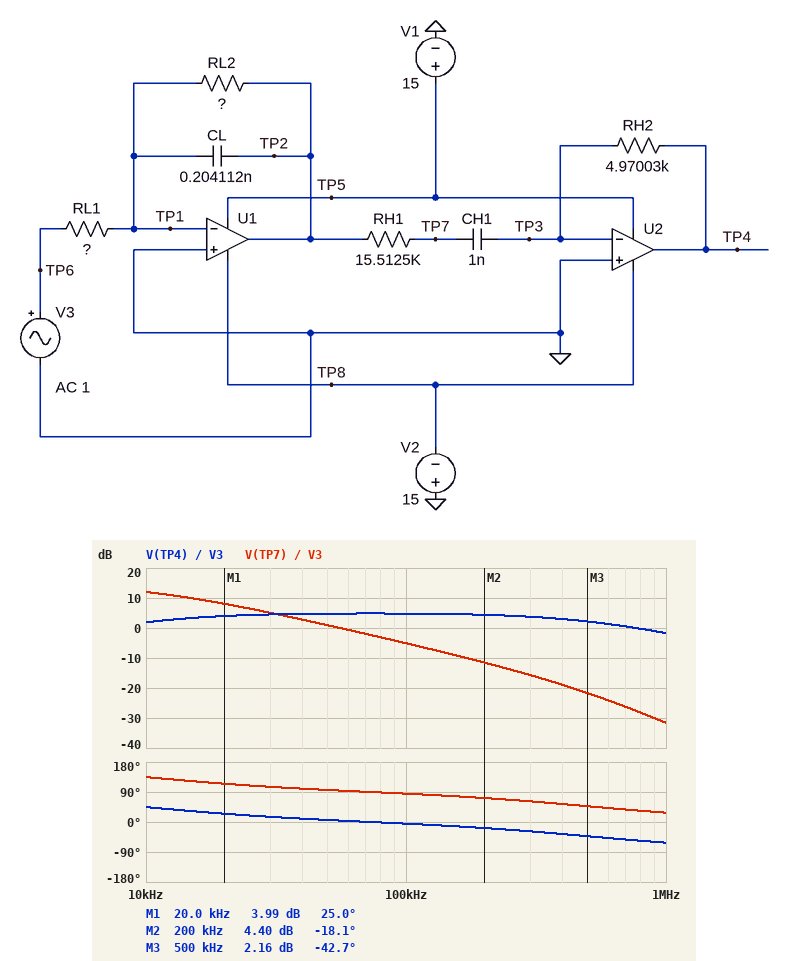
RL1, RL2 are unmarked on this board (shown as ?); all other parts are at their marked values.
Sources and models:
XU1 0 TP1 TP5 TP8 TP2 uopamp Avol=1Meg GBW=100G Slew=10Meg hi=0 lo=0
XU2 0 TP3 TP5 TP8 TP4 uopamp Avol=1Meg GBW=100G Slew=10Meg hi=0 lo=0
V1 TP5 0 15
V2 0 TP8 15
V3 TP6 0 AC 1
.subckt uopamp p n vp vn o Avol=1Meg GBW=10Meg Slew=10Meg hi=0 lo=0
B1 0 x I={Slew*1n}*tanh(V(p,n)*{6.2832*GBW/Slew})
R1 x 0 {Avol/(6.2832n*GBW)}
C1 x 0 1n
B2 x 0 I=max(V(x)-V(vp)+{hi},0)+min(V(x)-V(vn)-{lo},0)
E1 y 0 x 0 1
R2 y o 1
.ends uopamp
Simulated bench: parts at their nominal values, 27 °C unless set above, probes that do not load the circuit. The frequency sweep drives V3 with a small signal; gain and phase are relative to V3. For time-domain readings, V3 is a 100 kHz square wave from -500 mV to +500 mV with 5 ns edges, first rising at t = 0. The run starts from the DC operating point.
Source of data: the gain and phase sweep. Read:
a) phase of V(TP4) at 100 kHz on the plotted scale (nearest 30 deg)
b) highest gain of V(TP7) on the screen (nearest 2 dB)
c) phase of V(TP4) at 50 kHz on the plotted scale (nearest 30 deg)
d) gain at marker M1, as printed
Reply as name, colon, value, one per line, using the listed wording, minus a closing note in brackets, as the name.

phase of V(TP4) at 100 kHz on the plotted scale: 0 deg
highest gain of V(TP7) on the screen: 12 dB
phase of V(TP4) at 50 kHz on the plotted scale: 0 deg
gain at marker M1, as printed: 3.99 dB
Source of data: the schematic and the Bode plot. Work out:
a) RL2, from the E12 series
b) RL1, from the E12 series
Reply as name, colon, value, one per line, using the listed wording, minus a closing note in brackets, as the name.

RL2, from the E12 series: 1.5 kΩ
RL1, from the E12 series: 270 Ω
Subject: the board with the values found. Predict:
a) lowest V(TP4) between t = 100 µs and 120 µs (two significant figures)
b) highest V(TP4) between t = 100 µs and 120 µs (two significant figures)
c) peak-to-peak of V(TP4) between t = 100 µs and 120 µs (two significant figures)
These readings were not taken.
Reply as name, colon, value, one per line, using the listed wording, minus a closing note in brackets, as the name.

lowest V(TP4) between t = 100 µs and 120 µs: -940 mV
highest V(TP4) between t = 100 µs and 120 µs: 940 mV
peak-to-peak of V(TP4) between t = 100 µs and 120 µs: 1.9 V
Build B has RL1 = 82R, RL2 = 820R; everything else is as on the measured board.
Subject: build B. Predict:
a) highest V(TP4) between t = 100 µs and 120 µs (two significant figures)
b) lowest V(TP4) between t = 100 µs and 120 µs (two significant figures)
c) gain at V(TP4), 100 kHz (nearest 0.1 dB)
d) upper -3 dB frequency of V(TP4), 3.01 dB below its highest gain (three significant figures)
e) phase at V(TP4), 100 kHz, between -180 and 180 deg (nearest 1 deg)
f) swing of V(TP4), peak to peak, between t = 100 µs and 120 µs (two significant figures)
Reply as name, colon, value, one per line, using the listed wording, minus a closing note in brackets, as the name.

highest V(TP4) between t = 100 µs and 120 µs: 1.7 V
lowest V(TP4) between t = 100 µs and 120 µs: -1.7 V
gain at V(TP4), 100 kHz: 10.0 dB
upper -3 dB frequency of V(TP4), 3.01 dB below its highest gain: 971 kHz
phase at V(TP4), 100 kHz, between -180 and 180 deg: 0 deg
swing of V(TP4), peak to peak, between t = 100 µs and 120 µs: 3.5 V
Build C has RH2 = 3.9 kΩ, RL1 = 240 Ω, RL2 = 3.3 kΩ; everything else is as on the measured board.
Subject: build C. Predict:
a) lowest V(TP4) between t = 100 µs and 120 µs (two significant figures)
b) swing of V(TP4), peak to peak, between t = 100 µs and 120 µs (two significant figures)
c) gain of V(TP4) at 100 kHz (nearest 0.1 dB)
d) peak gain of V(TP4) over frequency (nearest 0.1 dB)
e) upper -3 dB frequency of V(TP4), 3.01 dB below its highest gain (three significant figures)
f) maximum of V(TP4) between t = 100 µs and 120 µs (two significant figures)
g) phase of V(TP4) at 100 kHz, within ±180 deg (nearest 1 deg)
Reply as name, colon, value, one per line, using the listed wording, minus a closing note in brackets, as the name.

lowest V(TP4) between t = 100 µs and 120 µs: -1.7 V
swing of V(TP4), peak to peak, between t = 100 µs and 120 µs: 3.4 V
gain of V(TP4) at 100 kHz: 10.0 dB
peak gain of V(TP4) over frequency: 10.4 dB
upper -3 dB frequency of V(TP4), 3.01 dB below its highest gain: 256 kHz
maximum of V(TP4) between t = 100 µs and 120 µs: 1.7 V
phase of V(TP4) at 100 kHz, within ±180 deg: -17 deg
